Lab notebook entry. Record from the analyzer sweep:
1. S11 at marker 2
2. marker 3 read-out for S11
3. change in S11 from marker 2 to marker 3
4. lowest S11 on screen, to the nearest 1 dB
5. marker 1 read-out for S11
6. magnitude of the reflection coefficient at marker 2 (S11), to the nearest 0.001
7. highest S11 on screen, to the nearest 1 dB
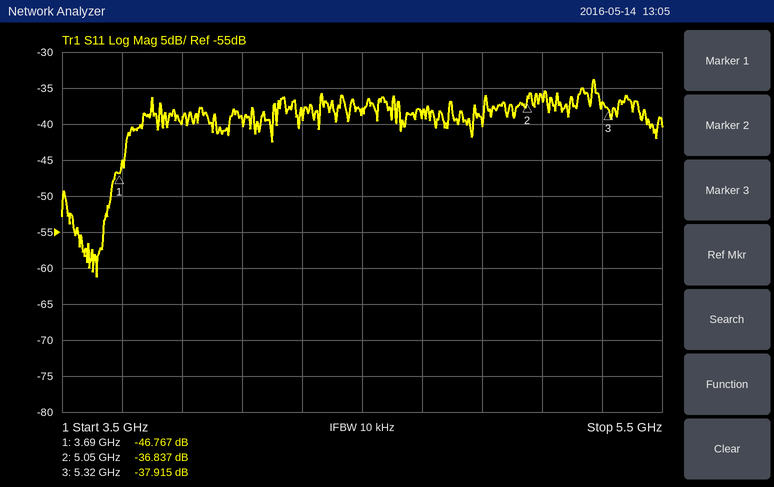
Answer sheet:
-36.837 dB
-37.915 dB
-1.078 dB
-61 dB
-46.767 dB
0.014
-34 dB
